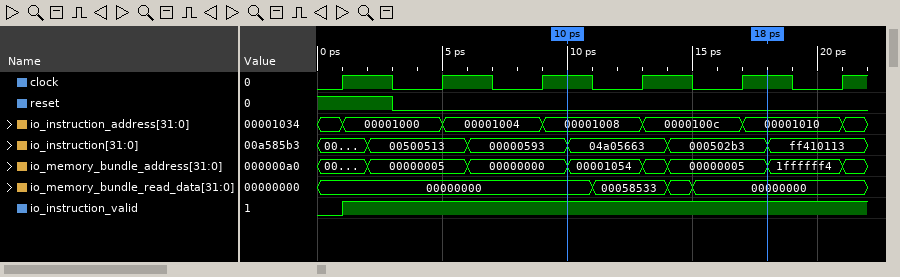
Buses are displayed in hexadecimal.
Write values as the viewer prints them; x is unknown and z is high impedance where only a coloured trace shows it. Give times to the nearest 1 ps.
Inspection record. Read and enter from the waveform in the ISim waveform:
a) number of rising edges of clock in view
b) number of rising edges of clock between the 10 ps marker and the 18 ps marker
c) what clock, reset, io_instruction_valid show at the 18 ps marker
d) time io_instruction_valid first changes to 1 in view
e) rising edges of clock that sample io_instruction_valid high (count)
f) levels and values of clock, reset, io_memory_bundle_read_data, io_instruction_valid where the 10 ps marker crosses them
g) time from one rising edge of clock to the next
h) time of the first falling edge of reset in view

6
2
clock=1, reset=0, io_instruction_valid=1
1 ps
5
clock=1, reset=0, io_memory_bundle_read_data=00000000, io_instruction_valid=1
4 ps
3 ps
